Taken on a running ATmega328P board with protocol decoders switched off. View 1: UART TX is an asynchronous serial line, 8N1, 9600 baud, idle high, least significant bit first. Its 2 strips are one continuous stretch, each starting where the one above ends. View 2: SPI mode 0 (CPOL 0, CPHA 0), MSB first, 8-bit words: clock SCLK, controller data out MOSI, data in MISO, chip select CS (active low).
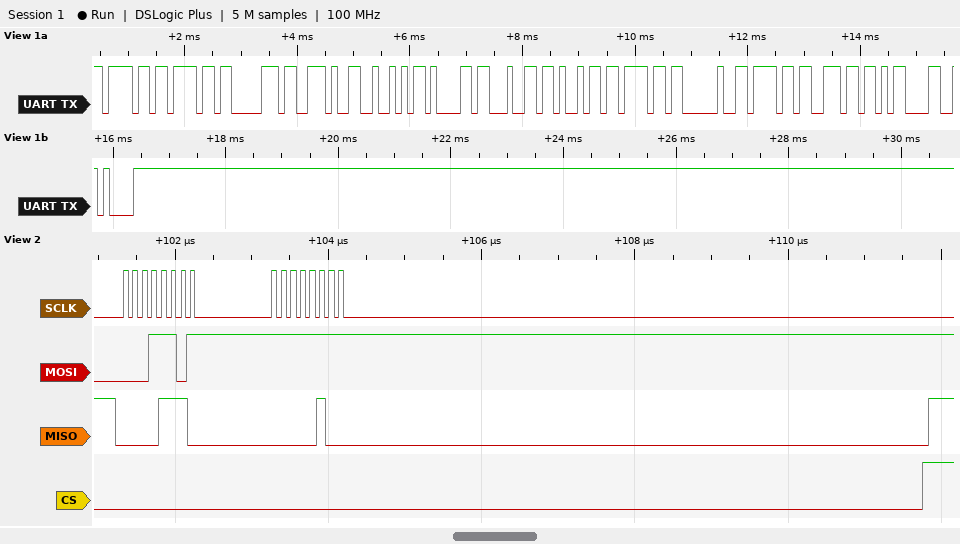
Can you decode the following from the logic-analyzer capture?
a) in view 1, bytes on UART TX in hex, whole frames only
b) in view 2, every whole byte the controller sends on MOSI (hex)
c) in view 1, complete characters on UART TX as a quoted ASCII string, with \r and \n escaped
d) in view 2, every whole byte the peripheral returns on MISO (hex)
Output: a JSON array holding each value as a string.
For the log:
["6F 6F 70 2E 52 61 64 69 6F 20 6F 6E 0D 0A", "1D FF", "\"oop.Radio on\\r\\n\"", "0E 04"]
